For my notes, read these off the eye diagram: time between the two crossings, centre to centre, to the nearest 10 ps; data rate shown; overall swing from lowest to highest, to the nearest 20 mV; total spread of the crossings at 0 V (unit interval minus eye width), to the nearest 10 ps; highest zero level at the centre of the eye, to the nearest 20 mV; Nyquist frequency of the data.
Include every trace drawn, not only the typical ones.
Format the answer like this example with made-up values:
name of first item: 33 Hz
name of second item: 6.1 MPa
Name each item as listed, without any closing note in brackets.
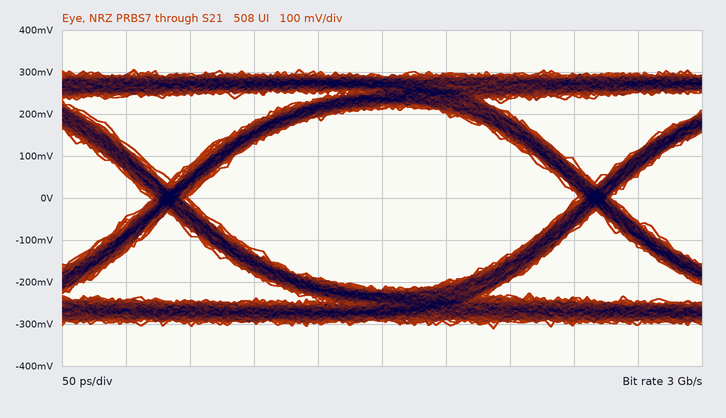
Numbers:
time between the two crossings, centre to centre, to the nearest 10 ps: 330 ps
data rate shown: 3 Gb/s
overall swing from lowest to highest, to the nearest 20 mV: 620 mV
total spread of the crossings at 0 V (unit interval minus eye width), to the nearest 10 ps: 30 ps
highest zero level at the centre of the eye, to the nearest 20 mV: -220 mV
Nyquist frequency of the data: 1.5 GHz
